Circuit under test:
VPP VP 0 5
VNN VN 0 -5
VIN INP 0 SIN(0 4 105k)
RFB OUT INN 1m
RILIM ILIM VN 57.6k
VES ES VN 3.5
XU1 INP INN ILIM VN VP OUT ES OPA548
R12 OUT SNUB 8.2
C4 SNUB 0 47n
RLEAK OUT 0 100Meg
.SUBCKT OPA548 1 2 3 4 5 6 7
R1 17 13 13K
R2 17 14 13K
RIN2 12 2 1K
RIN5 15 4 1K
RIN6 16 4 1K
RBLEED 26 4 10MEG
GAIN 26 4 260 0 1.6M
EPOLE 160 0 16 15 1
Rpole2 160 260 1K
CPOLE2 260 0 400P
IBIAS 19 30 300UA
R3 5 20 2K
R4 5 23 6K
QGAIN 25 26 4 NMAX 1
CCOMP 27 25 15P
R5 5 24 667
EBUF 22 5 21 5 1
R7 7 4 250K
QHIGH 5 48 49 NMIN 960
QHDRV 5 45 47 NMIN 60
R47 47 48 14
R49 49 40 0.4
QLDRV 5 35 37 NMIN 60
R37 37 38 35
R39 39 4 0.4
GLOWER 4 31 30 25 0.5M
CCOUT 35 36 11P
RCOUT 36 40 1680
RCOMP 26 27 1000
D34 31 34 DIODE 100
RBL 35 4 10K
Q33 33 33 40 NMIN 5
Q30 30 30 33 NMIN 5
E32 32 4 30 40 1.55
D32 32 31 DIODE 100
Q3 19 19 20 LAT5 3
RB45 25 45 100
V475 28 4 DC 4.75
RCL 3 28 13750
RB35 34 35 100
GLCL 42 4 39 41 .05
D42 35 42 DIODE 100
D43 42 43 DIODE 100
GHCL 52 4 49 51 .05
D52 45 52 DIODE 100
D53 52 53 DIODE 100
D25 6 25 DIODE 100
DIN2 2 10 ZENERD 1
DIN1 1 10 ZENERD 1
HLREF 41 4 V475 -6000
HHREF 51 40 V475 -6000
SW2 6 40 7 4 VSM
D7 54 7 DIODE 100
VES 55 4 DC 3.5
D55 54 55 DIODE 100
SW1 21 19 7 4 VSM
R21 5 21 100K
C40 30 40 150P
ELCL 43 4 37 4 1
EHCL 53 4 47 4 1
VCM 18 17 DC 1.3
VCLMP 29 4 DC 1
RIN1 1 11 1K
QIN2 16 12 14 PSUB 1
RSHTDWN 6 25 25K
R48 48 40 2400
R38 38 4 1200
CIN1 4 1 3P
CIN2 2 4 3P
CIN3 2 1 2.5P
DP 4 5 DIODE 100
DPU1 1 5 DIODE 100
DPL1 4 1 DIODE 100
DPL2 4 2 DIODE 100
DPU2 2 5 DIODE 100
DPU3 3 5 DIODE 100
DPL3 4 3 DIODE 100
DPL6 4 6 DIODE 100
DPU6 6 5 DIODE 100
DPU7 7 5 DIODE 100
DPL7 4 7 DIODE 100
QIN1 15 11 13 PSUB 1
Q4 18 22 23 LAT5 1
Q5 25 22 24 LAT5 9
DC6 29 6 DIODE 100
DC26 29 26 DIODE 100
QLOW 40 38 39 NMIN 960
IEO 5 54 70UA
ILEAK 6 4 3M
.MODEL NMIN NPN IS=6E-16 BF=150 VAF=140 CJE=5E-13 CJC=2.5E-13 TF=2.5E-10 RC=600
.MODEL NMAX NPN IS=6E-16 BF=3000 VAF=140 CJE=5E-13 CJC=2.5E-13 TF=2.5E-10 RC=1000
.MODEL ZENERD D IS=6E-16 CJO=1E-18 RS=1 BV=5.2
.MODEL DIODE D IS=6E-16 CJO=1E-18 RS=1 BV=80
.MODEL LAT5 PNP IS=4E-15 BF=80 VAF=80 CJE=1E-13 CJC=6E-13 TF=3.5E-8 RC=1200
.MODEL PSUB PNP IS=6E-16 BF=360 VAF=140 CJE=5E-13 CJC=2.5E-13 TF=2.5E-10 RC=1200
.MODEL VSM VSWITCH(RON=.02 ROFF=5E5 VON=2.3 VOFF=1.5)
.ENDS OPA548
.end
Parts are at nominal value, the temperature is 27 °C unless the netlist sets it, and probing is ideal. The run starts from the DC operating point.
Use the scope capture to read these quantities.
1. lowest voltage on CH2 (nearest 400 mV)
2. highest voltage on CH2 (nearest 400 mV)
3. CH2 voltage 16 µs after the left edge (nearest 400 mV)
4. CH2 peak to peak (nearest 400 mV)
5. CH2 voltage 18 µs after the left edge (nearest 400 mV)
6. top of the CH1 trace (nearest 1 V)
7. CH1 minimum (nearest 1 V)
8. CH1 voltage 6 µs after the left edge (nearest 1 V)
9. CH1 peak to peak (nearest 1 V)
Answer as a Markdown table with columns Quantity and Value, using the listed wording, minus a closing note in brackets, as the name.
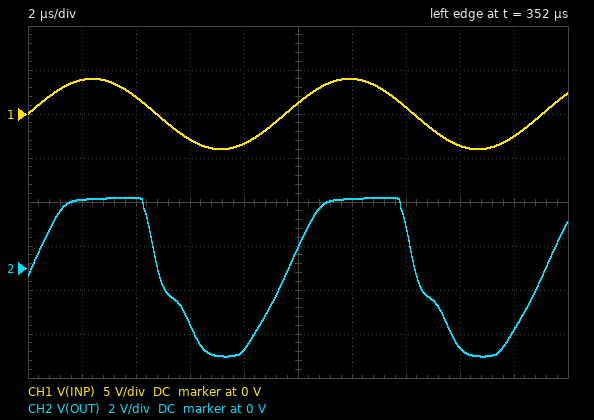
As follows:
| Quantity | Value |
|---|---|
| lowest voltage on CH2 | -4.0 V |
| highest voltage on CH2 | 3.2 V |
| CH2 voltage 16 µs after the left edge | -3.6 V |
| CH2 peak to peak | 7.2 V |
| CH2 voltage 18 µs after the left edge | -2.8 V |
| top of the CH1 trace | 4 V |
| CH1 minimum | -4 V |
| CH1 voltage 6 µs after the left edge | -3 V |
| CH1 peak to peak | 8 V |
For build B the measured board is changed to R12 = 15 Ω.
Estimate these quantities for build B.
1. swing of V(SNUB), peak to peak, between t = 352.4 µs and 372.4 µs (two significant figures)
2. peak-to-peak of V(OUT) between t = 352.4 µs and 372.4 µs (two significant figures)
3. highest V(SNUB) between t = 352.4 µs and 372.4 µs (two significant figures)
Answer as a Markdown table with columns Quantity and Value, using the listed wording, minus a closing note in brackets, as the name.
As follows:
| Quantity | Value |
|---|---|
| swing of V(SNUB), peak to peak, between t = 352.4 µs and 372.4 µs | 6.8 V |
| peak-to-peak of V(OUT) between t = 352.4 µs and 372.4 µs | 7.2 V |
| highest V(SNUB) between t = 352.4 µs and 372.4 µs | 3.1 V |
